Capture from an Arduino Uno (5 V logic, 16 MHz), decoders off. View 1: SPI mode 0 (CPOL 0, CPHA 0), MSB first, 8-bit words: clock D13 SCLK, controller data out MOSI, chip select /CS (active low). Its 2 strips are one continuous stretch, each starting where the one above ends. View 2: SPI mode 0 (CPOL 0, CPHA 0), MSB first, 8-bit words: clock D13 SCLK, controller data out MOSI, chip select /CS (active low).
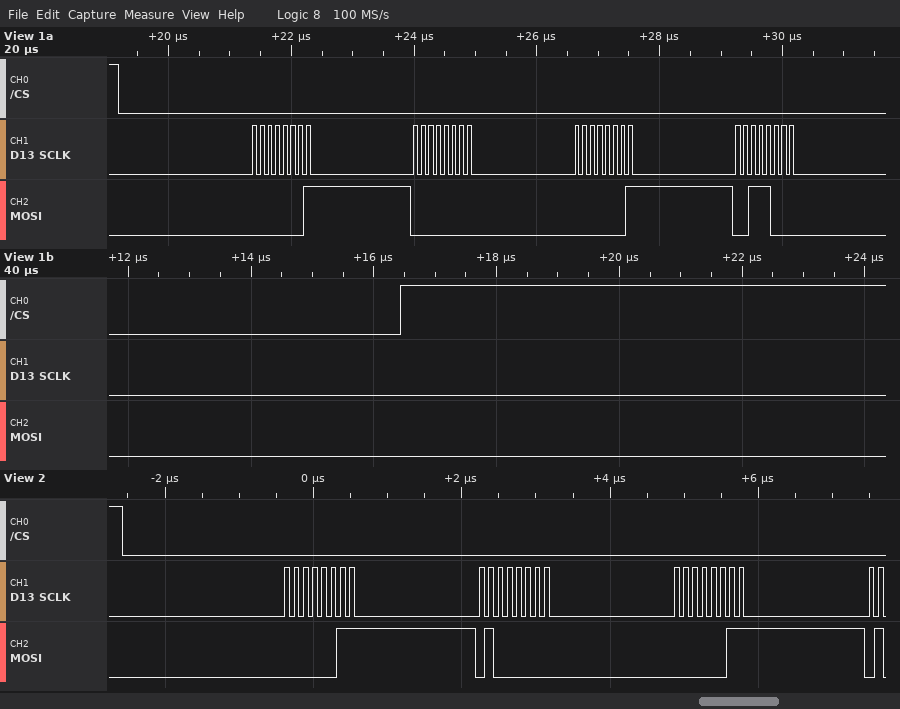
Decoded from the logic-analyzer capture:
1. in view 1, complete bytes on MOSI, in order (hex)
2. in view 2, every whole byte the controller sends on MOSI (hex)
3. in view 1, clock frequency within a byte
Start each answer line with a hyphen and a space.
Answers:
- 01 00 01 38
- 03 40 03
- 8 MHz
